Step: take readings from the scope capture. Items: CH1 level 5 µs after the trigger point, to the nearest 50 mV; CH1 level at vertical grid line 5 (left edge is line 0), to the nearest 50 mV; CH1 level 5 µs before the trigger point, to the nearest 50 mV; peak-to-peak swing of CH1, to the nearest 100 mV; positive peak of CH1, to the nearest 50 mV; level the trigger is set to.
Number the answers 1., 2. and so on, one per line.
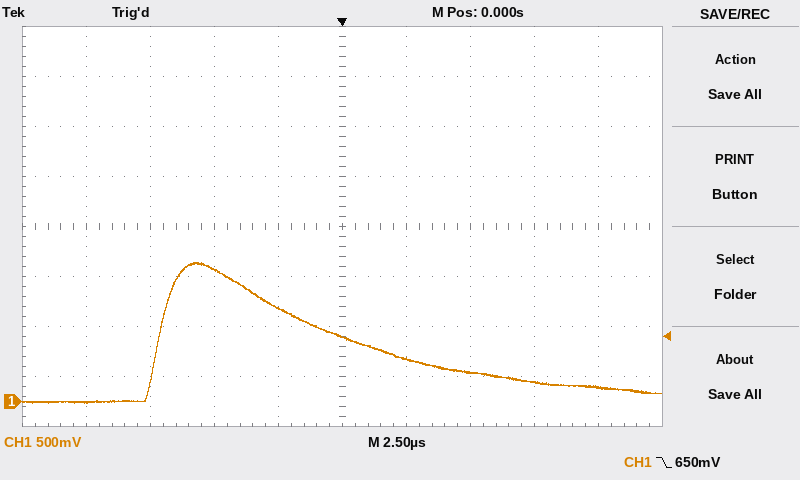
1. 300 mV
2. 650 mV
3. 1.30 V
4. 1.40 V
5. 1.40 V
6. 650 mV
